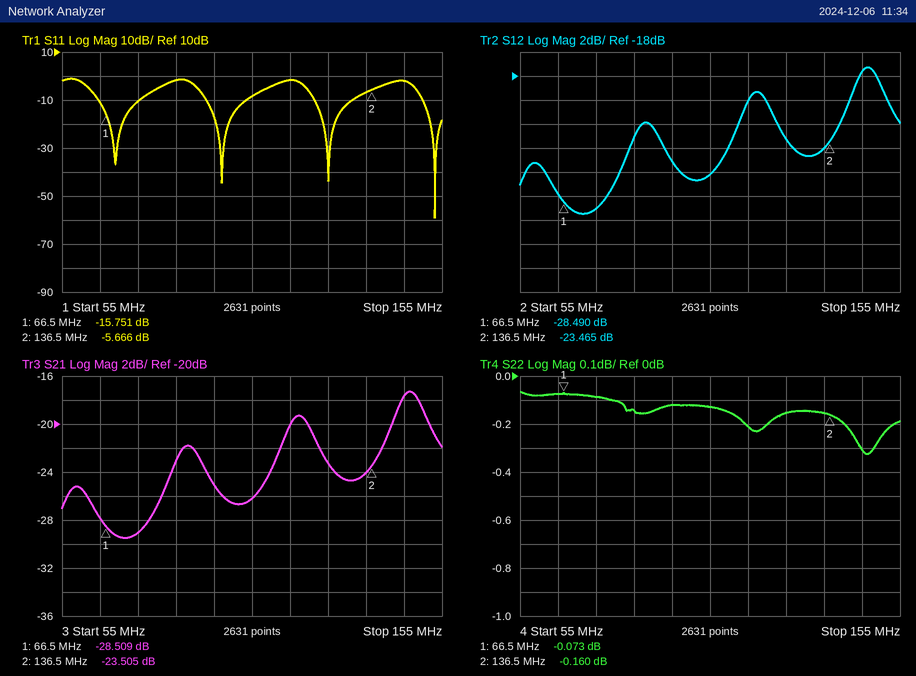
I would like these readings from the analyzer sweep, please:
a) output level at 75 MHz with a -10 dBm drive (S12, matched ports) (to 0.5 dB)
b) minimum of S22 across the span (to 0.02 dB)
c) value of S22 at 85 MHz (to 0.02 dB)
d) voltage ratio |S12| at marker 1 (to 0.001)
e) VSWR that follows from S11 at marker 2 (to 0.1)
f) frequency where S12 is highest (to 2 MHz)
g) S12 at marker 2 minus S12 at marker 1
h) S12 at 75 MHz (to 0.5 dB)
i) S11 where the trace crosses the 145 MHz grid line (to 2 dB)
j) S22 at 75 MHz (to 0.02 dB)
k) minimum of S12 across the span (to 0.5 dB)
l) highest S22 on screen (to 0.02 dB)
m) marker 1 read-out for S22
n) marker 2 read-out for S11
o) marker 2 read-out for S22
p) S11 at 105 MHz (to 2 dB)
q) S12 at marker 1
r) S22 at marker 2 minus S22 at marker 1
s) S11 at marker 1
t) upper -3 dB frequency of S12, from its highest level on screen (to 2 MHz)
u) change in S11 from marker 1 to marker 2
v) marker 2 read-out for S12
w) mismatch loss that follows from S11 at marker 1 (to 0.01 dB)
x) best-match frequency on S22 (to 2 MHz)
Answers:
-39.0 dBm
-0.32 dB
-0.14 dB
0.038
3.2
146 MHz
5.025 dB
-29.0 dB
-2 dB
-0.08 dB
-29.5 dB
-0.06 dB
-0.073 dB
-5.666 dB
-0.160 dB
-8 dB
-28.490 dB
-0.087 dB
-15.751 dB
152 MHz
10.085 dB
-23.465 dB
0.12 dB
146 MHz
